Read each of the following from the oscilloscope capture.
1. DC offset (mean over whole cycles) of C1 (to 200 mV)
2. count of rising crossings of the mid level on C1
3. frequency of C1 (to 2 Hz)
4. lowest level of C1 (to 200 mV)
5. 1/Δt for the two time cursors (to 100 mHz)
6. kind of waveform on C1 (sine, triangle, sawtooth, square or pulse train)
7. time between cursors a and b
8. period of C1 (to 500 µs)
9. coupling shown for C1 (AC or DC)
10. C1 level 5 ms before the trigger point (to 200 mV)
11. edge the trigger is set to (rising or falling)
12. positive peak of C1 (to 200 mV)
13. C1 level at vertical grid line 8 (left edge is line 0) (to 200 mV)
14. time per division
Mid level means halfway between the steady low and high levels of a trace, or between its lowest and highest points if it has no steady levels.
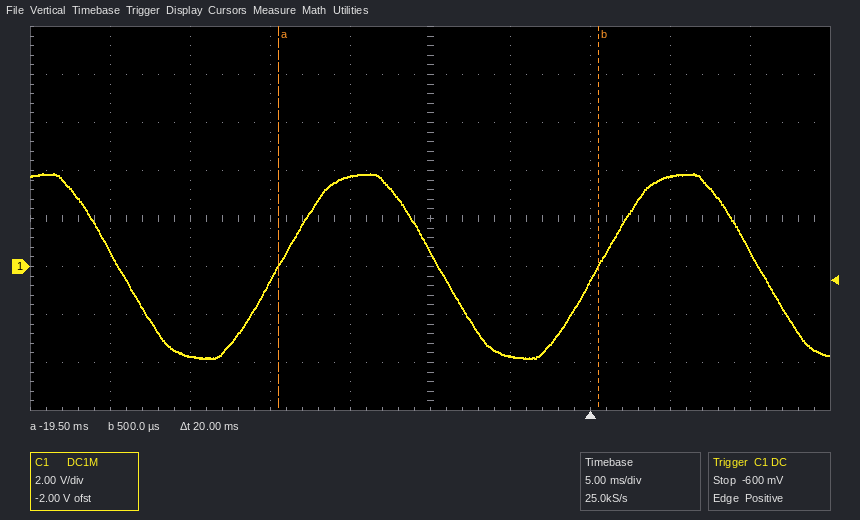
0.0 V
2
50 Hz
-3.8 V
50.0 Hz
sine
20 ms
20.0 ms
DC
-3.8 V
rising
3.8 V
3.8 V
5 ms
